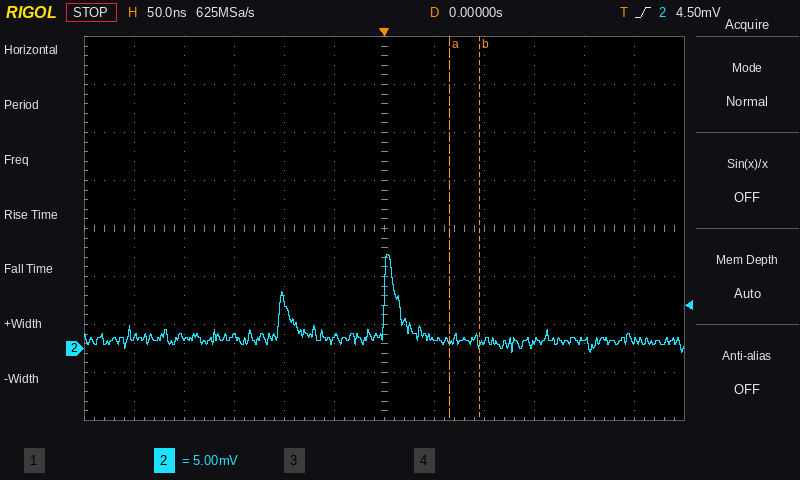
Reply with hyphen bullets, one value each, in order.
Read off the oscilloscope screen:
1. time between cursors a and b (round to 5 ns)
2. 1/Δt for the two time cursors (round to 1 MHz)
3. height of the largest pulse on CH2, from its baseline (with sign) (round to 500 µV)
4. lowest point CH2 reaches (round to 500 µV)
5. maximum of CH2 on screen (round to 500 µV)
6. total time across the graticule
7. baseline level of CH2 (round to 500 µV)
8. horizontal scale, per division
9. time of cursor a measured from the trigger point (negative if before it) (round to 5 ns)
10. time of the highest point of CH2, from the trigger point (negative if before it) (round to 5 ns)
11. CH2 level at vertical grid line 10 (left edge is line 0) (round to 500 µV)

- 30 ns
- 33 MHz
- +9.0 mV
- -500 µV
- 10.0 mV
- 600 ns
- 1.0 mV
- 50 ns
- +65 ns
- +5 ns
- 1.0 mV
